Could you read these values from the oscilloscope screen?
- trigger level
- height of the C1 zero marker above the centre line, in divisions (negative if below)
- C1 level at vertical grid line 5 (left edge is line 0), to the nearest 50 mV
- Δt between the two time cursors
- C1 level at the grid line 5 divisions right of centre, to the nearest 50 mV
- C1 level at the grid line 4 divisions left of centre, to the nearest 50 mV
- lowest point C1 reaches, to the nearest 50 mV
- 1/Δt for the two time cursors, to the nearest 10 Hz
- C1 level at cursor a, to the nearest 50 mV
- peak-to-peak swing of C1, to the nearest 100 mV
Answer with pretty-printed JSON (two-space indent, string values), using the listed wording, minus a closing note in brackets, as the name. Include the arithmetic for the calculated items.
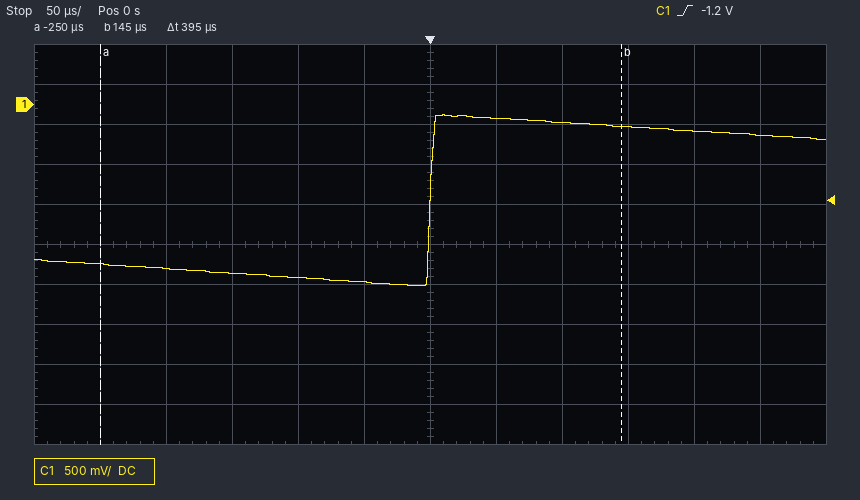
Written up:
{
  "trigger level": "-1.2 V",
  "height of the C1 zero marker above the centre line, in divisions": "+3.5 div",
  "C1 level at vertical grid line 5 (left edge is line 0), to the nearest 50 mV": "-2.20 V",
  "Δt between the two time cursors": "395 µs",
  "C1 level at the grid line 5 divisions right of centre, to the nearest 50 mV": "-400 mV",
  "C1 level at the grid line 4 divisions left of centre, to the nearest 50 mV": "-2.05 V",
  "lowest point C1 reaches, to the nearest 50 mV": "-2.25 V",
  "1/Δt for the two time cursors, to the nearest 10 Hz": "1 / 395 µs ≈ 2.53 kHz",
  "C1 level at cursor a, to the nearest 50 mV": "-2.00 V",
  "peak-to-peak swing of C1, to the nearest 100 mV": "2.10 V"
}
